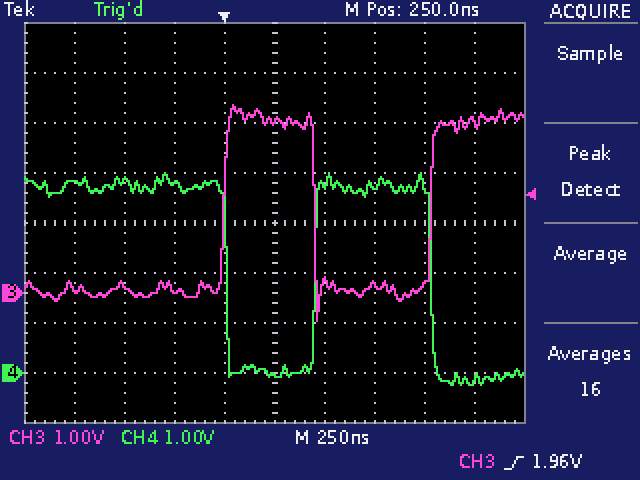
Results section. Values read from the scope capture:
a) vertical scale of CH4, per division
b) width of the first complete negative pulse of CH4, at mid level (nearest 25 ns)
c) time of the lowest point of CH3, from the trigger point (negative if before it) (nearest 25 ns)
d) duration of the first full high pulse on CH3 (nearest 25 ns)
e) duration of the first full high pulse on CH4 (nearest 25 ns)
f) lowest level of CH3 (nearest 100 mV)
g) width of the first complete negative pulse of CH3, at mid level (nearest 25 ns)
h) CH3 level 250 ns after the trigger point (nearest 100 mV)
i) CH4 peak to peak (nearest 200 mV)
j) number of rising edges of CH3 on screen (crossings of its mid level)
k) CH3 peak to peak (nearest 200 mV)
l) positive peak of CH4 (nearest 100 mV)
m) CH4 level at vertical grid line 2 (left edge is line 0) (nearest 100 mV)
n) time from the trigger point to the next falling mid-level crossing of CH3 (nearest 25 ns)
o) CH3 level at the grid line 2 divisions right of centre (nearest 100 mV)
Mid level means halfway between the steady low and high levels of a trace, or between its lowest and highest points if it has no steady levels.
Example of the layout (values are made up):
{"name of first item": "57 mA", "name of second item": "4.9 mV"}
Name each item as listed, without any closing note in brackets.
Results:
{"vertical scale of CH4, per division": "1 V", "width of the first complete negative pulse of CH4, at mid level": "450 ns", "time of the lowest point of CH3, from the trigger point (negative if before it)": "+475 ns", "duration of the first full high pulse on CH3": "450 ns", "duration of the first full high pulse on CH4": "575 ns", "lowest level of CH3": "-600 mV", "width of the first complete negative pulse of CH3, at mid level": "575 ns", "CH3 level 250 ns after the trigger point": "3.4 V", "CH4 peak to peak": "4.2 V", "number of rising edges of CH3 on screen": "2", "CH3 peak to peak": "4.4 V", "positive peak of CH4": "4.0 V", "CH4 level at vertical grid line 2 (left edge is line 0)": "3.8 V", "time from the trigger point to the next falling mid-level crossing of CH3": "450 ns", "CH3 level at the grid line 2 divisions right of centre": "200 mV"}
